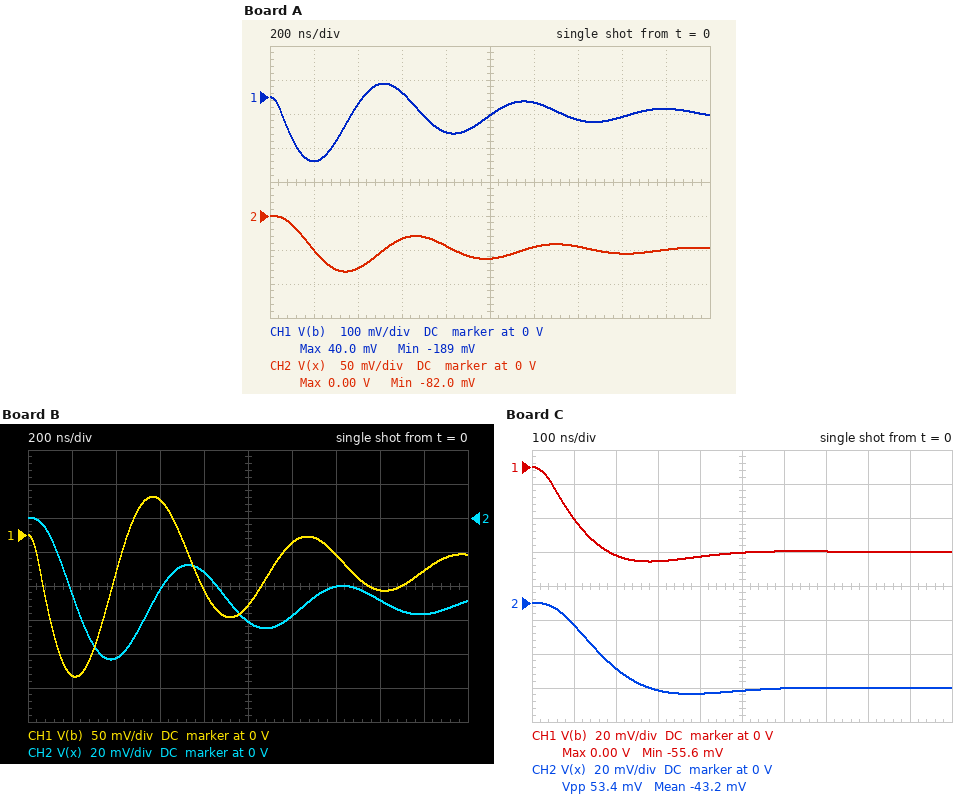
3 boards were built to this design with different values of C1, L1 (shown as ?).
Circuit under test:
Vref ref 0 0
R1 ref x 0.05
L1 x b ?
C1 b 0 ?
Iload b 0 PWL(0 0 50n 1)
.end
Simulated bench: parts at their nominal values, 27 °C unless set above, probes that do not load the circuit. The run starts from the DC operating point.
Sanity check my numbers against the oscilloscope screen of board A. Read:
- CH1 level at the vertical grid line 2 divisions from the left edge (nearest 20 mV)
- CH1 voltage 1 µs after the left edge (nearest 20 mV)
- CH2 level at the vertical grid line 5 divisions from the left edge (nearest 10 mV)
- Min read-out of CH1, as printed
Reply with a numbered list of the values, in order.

1. -20 mV
2. -60 mV
3. -60 mV
4. -189 mV
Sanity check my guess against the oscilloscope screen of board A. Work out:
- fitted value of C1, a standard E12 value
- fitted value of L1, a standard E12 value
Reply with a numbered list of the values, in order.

1. 560 nF
2. 18 nH
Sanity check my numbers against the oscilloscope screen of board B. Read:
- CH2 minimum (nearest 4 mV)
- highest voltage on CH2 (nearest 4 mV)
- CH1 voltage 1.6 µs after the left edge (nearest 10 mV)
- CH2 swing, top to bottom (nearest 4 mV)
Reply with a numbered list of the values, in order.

1. -84 mV
2. 0 V
3. -80 mV
4. 84 mV
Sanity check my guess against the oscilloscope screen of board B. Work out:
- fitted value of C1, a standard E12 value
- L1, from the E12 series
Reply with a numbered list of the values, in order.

1. 560 nF
2. 22 nH
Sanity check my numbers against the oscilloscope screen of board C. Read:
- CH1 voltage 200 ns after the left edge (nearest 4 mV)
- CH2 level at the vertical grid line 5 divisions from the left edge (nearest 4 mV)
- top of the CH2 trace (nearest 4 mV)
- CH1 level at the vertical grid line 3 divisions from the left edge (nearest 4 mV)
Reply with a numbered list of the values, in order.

1. -52 mV
2. -52 mV
3. 0 V
4. -56 mV
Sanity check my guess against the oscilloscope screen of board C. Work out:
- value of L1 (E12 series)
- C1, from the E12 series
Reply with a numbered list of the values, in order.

1. 3.3 nH
2. 2.2 µF
